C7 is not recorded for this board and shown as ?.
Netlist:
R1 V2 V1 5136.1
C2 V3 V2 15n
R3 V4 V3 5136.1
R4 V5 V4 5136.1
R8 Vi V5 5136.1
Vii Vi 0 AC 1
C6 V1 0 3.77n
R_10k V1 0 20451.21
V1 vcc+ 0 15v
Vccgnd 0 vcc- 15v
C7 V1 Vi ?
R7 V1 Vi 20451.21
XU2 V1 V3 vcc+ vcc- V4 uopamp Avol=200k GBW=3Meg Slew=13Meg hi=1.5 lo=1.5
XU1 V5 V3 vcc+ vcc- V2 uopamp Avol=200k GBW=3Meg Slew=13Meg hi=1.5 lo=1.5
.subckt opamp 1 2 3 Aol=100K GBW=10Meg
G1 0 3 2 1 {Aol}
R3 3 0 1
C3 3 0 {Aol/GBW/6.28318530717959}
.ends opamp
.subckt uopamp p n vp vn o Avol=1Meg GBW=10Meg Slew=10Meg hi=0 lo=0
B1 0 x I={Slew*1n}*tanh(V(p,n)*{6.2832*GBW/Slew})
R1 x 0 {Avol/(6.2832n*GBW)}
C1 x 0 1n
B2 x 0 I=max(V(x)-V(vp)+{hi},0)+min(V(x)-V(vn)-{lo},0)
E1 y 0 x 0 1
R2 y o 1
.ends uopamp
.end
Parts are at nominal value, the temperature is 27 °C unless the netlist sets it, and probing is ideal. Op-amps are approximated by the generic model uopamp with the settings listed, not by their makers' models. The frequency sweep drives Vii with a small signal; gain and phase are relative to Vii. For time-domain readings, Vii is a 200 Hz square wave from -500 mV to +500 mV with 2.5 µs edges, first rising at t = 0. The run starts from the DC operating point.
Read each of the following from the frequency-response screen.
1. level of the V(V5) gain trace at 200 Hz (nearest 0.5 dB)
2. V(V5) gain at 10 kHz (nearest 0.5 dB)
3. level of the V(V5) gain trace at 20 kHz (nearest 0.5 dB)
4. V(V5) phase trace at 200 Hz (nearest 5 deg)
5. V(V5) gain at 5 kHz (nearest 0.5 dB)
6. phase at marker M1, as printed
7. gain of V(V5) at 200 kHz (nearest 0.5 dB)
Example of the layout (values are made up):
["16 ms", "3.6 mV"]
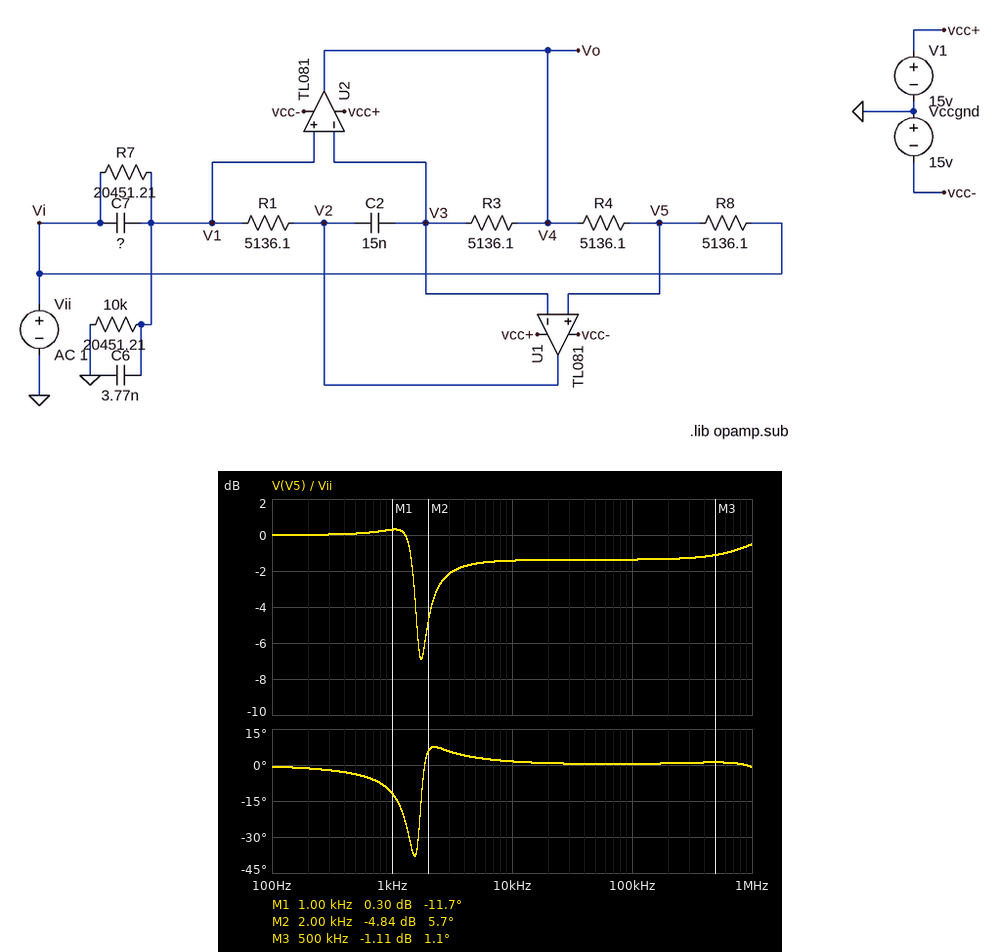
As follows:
["0 dB", "-1.5 dB", "-1.5 dB", "0 deg", "-1.5 dB", "-11.7 deg", "-1.5 dB"]
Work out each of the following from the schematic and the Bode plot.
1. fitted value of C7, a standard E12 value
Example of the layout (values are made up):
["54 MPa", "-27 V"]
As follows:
["22 nF"]
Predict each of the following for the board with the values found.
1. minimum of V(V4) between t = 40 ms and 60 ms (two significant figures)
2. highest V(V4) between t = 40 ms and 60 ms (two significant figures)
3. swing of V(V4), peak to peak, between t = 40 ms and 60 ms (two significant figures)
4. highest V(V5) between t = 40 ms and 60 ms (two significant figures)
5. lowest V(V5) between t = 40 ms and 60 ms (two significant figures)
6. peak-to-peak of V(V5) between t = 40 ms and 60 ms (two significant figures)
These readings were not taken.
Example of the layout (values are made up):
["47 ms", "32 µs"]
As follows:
["-710 mV", "710 mV", "1.4 V", "600 mV", "-600 mV", "1.2 V"]
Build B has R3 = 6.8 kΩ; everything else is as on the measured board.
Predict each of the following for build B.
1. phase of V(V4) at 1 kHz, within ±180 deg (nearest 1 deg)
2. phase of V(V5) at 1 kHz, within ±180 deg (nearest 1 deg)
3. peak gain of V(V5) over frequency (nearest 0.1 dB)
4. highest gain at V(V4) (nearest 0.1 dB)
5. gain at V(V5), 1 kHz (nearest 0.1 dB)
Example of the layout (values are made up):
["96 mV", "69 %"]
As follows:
["-35 deg", "-18 deg", "0.2 dB", "0.8 dB", "0 dB"]
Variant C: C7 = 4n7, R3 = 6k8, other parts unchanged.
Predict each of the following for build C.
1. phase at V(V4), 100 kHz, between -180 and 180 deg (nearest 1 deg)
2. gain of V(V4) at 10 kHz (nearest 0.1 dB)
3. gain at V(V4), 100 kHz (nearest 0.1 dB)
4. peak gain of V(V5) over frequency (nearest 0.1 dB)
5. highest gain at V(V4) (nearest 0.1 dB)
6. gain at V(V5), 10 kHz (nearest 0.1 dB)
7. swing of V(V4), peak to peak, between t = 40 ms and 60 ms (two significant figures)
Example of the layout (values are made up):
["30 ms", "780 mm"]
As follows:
["16 deg", "-25.0 dB", "-18.7 dB", "0.5 dB", "2.3 dB", "-5.6 dB", "1.5 V"]
